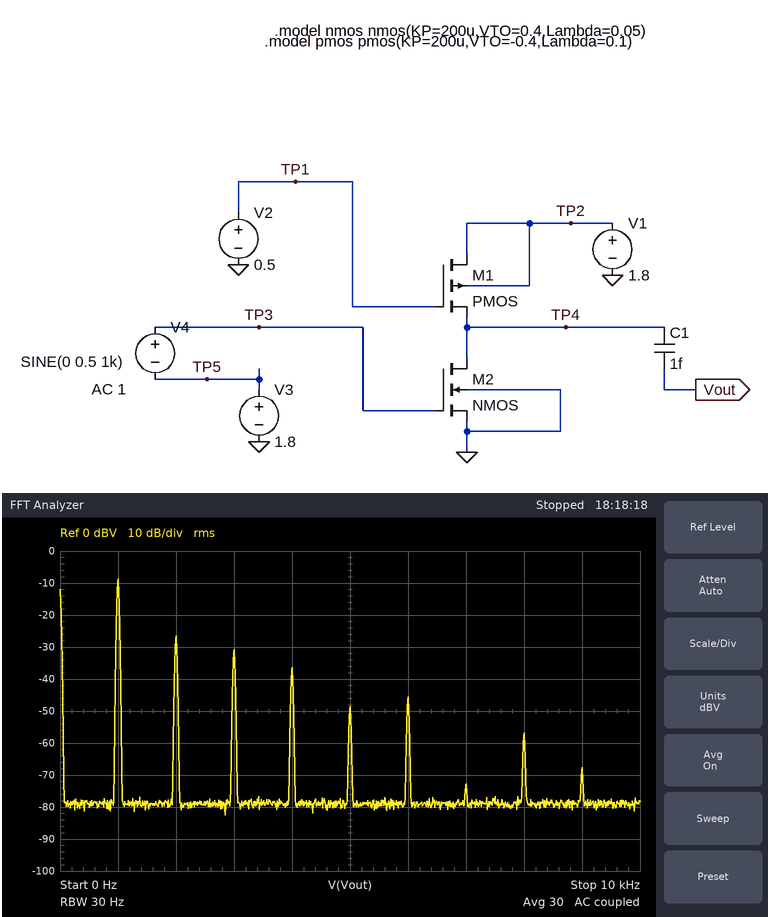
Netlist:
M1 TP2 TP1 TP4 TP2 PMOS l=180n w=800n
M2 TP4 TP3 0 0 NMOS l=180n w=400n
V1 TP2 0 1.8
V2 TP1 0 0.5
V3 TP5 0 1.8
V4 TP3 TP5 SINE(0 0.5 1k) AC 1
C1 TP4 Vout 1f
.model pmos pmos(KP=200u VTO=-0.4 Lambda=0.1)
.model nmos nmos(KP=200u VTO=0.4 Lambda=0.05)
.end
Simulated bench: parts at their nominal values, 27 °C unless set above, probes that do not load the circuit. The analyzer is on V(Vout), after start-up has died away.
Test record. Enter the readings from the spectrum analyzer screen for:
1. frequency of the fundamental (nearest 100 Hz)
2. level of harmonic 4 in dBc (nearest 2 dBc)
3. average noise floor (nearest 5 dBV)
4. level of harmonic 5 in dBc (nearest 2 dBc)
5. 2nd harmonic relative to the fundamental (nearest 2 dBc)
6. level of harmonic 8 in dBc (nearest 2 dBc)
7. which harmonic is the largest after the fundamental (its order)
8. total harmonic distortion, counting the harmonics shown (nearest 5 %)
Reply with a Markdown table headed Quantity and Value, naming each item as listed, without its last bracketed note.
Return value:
| Quantity | Value |
|---|---|
| frequency of the fundamental | 1.0 kHz |
| level of harmonic 4 in dBc | -28 dBc |
| average noise floor | -80 dBV |
| level of harmonic 5 in dBc | -40 dBc |
| 2nd harmonic relative to the fundamental | -18 dBc |
| level of harmonic 8 in dBc | -48 dBc |
| which harmonic is the largest after the fundamental | 2 |
| total harmonic distortion, counting the harmonics shown | 15 % |
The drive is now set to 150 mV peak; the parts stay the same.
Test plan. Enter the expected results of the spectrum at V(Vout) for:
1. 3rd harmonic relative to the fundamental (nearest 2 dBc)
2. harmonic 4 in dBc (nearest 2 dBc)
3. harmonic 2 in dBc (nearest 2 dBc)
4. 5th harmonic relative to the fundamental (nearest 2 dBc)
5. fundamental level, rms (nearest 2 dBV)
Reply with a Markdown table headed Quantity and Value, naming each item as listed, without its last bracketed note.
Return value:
| Quantity | Value |
|---|---|
| 3rd harmonic relative to the fundamental | -38 dBc |
| harmonic 4 in dBc | -44 dBc |
| harmonic 2 in dBc | -20 dBc |
| 5th harmonic relative to the fundamental | -50 dBc |
| fundamental level, rms | -18 dBV |
